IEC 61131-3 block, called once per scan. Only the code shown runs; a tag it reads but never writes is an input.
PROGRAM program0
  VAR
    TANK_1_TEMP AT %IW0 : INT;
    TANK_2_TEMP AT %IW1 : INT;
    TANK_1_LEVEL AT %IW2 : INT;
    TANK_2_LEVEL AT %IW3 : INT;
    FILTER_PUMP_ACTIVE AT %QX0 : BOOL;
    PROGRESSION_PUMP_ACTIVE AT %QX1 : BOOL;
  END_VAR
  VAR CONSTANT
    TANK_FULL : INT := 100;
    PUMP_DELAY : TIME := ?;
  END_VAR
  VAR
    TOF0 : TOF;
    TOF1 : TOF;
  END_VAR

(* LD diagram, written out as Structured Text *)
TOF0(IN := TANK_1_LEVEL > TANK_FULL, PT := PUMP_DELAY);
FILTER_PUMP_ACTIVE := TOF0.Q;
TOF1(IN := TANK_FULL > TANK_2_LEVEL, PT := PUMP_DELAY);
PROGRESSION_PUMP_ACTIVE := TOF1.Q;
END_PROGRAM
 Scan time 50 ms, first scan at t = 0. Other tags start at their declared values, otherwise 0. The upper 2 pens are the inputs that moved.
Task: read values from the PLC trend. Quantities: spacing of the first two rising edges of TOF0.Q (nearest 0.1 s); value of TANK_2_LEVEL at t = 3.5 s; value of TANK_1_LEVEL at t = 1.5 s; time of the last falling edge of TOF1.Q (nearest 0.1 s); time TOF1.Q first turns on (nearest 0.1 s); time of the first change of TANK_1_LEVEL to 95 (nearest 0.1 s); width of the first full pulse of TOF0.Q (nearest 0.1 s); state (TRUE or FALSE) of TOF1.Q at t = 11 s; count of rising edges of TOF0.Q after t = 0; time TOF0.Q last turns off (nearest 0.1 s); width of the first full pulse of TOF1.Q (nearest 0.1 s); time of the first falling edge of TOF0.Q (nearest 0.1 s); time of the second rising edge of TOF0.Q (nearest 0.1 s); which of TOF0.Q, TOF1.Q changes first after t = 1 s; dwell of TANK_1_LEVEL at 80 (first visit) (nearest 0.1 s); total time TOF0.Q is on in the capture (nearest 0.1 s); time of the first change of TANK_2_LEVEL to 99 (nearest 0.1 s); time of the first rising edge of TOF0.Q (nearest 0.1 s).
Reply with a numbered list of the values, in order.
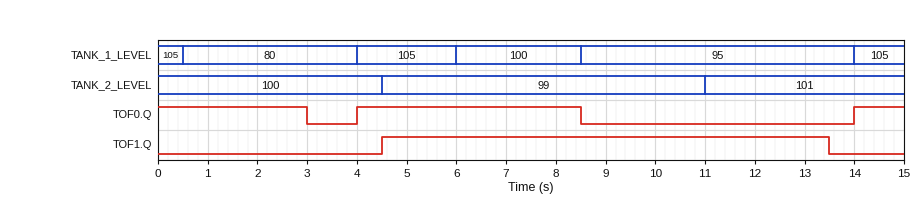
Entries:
1. 10.0 s
2. 100
3. 80
4. 13.5 s
5. 4.5 s
6. 8.5 s
7. 4.5 s
8. TRUE
9. 2
10. 8.5 s
11. 9.0 s
12. 3.0 s
13. 14.0 s
14. TOF0.Q
15. 3.5 s
16. 8.5 s
17. 4.5 s
18. 4.0 s
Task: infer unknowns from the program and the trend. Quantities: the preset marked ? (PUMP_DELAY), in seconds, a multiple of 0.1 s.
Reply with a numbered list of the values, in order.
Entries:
1. 2.5 s
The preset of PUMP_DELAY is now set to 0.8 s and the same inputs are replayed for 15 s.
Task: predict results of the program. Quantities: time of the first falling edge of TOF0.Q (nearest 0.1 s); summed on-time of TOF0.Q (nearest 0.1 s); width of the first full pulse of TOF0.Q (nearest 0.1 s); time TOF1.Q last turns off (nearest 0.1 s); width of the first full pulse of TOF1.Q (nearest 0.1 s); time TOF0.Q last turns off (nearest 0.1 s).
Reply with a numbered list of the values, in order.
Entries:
1. 1.3 s
2. 5.1 s
3. 2.8 s
4. 11.8 s
5. 7.3 s
6. 6.8 s
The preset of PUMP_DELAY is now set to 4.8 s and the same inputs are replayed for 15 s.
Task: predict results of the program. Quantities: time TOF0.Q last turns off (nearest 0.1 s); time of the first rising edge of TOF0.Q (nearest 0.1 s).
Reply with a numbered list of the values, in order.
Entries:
1. 10.8 s
2. 14.0 s
